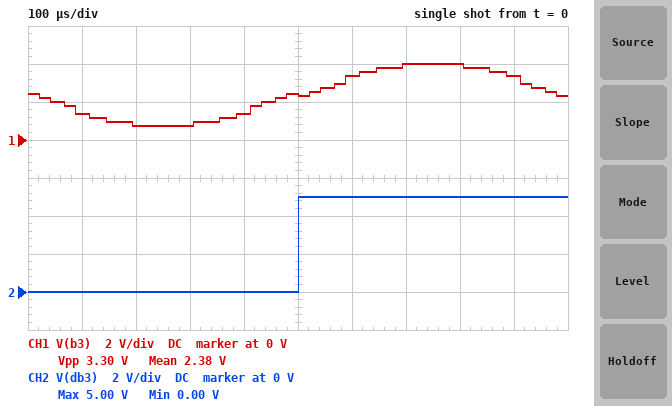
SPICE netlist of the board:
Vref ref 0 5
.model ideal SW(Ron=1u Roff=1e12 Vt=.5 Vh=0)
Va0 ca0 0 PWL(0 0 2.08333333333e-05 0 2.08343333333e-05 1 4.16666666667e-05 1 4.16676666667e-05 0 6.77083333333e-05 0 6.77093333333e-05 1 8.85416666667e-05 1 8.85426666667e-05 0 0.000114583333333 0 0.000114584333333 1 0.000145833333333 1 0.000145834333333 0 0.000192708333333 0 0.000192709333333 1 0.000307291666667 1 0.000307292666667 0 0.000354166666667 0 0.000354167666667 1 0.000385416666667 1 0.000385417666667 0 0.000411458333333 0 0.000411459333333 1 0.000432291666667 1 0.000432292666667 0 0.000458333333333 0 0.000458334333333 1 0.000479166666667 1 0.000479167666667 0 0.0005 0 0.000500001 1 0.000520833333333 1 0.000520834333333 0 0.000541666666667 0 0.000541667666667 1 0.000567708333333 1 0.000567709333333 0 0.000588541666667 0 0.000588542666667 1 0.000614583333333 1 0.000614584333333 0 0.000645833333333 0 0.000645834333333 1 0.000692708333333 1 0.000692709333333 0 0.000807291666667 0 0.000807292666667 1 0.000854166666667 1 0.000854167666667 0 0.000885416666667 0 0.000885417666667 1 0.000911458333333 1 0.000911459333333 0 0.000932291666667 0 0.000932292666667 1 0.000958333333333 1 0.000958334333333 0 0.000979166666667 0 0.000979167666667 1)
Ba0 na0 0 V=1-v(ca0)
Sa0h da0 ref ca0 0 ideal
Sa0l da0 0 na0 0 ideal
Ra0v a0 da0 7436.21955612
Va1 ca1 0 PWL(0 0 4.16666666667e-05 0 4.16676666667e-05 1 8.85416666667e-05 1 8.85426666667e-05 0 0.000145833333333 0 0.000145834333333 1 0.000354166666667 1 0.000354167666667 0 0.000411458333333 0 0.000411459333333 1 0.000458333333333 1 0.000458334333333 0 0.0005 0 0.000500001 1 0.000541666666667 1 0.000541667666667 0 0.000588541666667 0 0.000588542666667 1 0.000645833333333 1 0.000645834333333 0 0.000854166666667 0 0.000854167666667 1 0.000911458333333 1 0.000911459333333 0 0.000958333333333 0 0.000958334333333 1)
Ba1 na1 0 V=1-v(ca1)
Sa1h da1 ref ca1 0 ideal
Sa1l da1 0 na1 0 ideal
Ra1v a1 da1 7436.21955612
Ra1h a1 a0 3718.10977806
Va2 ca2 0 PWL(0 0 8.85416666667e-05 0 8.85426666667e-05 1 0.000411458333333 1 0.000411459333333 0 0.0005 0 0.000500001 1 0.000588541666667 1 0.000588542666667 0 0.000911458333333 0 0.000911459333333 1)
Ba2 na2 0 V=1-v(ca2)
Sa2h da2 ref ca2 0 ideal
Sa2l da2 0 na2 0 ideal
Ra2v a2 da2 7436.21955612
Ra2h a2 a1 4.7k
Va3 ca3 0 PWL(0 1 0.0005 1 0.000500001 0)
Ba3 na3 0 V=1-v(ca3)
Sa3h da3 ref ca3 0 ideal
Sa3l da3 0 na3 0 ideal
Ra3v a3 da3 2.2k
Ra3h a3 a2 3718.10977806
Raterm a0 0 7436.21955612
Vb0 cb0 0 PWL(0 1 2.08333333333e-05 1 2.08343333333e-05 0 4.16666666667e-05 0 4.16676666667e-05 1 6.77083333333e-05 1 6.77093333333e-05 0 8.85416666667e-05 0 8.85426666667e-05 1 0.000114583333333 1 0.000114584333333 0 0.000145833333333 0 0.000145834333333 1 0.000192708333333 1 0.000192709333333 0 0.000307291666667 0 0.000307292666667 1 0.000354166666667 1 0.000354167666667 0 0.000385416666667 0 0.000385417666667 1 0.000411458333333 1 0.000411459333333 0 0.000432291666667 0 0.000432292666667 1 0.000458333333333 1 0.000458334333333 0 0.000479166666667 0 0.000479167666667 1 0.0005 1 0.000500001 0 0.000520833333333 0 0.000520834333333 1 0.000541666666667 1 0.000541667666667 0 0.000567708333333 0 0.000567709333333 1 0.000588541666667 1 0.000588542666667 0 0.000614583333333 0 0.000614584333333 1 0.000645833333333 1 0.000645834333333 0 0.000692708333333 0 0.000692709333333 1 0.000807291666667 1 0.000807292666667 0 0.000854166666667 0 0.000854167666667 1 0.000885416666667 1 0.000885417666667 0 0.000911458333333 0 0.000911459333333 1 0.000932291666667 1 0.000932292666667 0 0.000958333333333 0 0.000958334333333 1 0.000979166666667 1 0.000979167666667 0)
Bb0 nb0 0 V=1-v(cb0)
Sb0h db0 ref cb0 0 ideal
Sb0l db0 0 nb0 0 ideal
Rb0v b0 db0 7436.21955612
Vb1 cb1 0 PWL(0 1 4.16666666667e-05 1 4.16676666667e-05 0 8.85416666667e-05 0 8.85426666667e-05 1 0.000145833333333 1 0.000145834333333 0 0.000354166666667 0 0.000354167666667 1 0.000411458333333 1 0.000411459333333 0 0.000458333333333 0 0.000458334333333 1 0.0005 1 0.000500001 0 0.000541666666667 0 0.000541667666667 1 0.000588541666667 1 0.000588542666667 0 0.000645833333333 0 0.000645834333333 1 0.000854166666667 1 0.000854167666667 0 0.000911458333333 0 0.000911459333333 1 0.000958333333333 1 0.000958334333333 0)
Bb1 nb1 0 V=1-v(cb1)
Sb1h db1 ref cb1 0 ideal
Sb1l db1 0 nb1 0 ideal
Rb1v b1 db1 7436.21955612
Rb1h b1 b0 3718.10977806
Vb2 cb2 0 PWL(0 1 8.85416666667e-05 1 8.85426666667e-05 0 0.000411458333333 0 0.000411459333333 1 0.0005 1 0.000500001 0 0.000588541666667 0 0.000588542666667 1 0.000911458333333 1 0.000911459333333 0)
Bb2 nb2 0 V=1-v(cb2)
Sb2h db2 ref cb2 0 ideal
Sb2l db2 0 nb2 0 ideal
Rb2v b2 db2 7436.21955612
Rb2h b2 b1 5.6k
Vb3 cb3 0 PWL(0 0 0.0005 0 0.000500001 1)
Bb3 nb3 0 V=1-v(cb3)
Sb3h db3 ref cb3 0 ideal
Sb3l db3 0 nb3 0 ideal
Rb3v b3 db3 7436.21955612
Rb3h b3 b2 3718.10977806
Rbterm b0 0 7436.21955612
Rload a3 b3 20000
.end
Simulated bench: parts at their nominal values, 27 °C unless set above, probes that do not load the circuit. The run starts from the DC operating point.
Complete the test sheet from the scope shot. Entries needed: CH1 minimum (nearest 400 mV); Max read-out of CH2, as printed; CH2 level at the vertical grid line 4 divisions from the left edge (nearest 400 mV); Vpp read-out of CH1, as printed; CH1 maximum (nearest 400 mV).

800 mV
5.00 V
0 V
3.30 V
4.0 V
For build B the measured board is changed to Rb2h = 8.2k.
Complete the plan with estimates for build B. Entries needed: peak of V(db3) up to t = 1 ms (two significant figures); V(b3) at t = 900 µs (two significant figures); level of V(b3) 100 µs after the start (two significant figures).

5.0 V
3.5 V
1.3 V
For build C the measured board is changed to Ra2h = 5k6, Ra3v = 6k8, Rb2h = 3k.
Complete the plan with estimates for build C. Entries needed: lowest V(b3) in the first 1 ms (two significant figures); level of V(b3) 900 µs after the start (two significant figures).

640 mV
3.3 V
